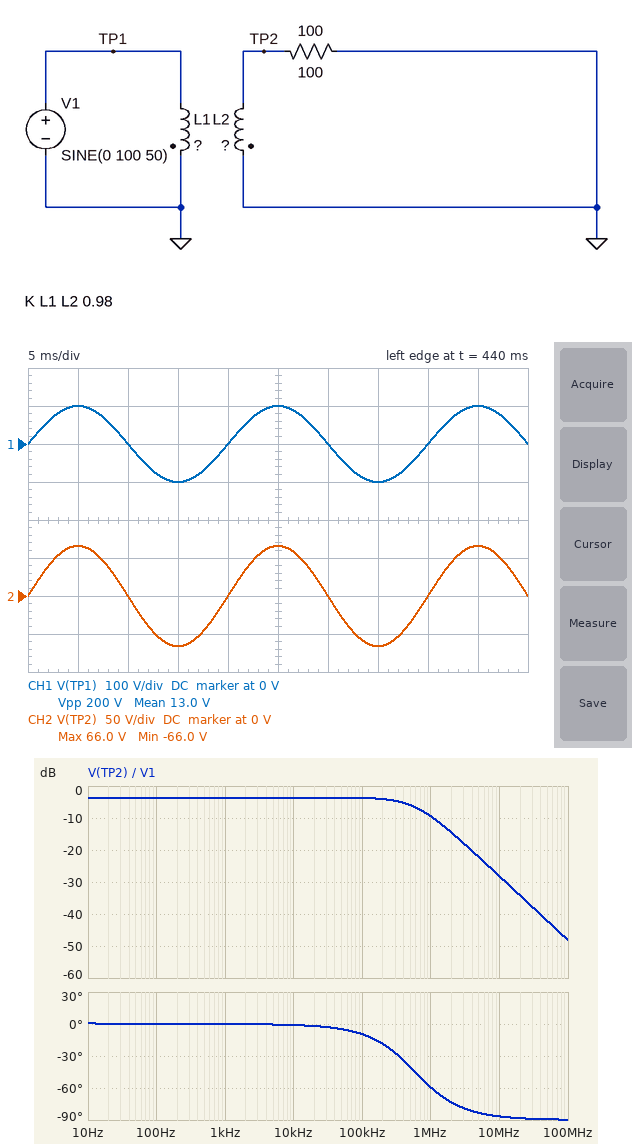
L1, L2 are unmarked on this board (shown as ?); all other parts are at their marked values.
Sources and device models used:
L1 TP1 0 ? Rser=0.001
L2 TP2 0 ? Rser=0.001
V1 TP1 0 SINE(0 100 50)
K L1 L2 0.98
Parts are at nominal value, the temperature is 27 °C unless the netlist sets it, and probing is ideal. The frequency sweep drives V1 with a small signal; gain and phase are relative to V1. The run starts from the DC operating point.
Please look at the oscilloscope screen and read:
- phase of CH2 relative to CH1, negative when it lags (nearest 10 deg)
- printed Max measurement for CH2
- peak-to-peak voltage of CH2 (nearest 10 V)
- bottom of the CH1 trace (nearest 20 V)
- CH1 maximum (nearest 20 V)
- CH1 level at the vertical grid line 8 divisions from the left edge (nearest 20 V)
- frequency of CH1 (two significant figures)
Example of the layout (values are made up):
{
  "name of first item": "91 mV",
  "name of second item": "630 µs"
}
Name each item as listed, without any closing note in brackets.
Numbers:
{
  "phase of CH2 relative to CH1, negative when it lags": "0 deg",
  "printed Max measurement for CH2": "66.0 V",
  "peak-to-peak voltage of CH2": "130 V",
  "bottom of the CH1 trace": "-100 V",
  "CH1 maximum": "100 V",
  "CH1 level at the vertical grid line 8 divisions from the left edge": "0 V",
  "frequency of CH1": "50 Hz"
}
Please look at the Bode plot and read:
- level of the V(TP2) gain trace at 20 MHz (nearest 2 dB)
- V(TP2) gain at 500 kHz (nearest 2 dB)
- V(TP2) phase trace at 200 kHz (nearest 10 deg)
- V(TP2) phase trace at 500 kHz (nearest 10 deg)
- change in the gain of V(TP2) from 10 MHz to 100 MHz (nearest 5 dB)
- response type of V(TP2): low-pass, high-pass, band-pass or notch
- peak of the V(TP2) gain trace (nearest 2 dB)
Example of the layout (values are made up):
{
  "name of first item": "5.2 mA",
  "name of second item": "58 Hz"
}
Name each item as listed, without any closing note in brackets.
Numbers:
{
  "level of the V(TP2) gain trace at 20 MHz": "-34 dB",
  "V(TP2) gain at 500 kHz": "-6 dB",
  "V(TP2) phase trace at 200 kHz": "-20 deg",
  "V(TP2) phase trace at 500 kHz": "-40 deg",
  "change in the gain of V(TP2) from 10 MHz to 100 MHz": "-20 dB",
  "response type of V(TP2): low-pass, high-pass, band-pass or notch": "low-pass",
  "peak of the V(TP2) gain trace": "-4 dB"
}
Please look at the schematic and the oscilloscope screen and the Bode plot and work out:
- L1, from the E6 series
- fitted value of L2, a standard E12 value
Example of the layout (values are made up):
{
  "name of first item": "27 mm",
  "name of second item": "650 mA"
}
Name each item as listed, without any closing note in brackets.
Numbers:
{
  "L1, from the E6 series": "1.5 mH",
  "fitted value of L2, a standard E12 value": "680 µH"
}
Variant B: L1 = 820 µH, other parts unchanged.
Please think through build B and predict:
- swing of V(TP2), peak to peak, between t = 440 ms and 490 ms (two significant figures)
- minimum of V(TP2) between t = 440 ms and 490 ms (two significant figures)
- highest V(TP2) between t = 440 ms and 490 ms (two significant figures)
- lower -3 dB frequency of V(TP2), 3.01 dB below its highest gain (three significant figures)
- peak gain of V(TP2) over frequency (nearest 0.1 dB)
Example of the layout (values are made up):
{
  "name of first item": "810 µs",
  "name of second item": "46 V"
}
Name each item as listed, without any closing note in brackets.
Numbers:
{
  "swing of V(TP2), peak to peak, between t = 440 ms and 490 ms": "180 V",
  "minimum of V(TP2) between t = 440 ms and 490 ms": "-89 V",
  "highest V(TP2) between t = 440 ms and 490 ms": "89 V",
  "lower -3 dB frequency of V(TP2), 3.01 dB below its highest gain": "194 mHz",
  "peak gain of V(TP2) over frequency": "-1.0 dB"
}
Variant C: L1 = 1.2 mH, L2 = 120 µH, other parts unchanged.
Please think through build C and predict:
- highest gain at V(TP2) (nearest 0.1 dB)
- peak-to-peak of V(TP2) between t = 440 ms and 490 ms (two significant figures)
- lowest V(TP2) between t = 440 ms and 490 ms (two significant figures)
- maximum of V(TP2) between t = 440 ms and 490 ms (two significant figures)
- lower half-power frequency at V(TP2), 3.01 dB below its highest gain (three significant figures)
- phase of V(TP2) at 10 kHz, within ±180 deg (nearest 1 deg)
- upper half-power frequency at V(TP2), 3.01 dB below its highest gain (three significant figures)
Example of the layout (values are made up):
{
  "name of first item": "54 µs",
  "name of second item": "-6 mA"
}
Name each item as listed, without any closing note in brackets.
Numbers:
{
  "highest gain at V(TP2)": "-10.2 dB",
  "peak-to-peak of V(TP2) between t = 440 ms and 490 ms": "62 V",
  "lowest V(TP2) between t = 440 ms and 490 ms": "-31 V",
  "maximum of V(TP2) between t = 440 ms and 490 ms": "31 V",
  "lower half-power frequency at V(TP2), 3.01 dB below its highest gain": "133 mHz",
  "phase of V(TP2) at 10 kHz, within ±180 deg": "0 deg",
  "upper half-power frequency at V(TP2), 3.01 dB below its highest gain": "3.35 MHz"
}
